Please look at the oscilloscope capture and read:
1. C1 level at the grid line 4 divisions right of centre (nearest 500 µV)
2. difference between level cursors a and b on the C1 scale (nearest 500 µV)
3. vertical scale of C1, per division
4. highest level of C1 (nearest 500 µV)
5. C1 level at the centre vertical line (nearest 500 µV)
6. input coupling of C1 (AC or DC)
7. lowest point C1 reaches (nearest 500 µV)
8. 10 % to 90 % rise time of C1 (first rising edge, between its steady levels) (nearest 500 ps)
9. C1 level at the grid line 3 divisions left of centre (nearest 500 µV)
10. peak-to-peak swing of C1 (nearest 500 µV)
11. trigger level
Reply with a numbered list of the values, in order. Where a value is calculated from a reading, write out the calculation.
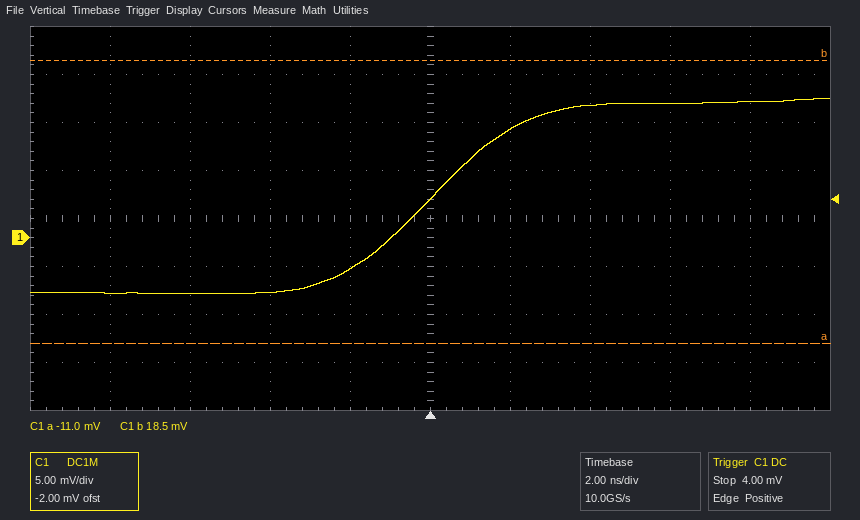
1. 14.0 mV
2. 29.5 mV
3. 5 mV
4. 14.5 mV
5. 4.0 mV
6. DC
7. -6.0 mV
8. 4.5 ns
9. -6.0 mV
10. 14.5 mV − (-6.0 mV) = 20.5 mV
11. 4.00 mV
